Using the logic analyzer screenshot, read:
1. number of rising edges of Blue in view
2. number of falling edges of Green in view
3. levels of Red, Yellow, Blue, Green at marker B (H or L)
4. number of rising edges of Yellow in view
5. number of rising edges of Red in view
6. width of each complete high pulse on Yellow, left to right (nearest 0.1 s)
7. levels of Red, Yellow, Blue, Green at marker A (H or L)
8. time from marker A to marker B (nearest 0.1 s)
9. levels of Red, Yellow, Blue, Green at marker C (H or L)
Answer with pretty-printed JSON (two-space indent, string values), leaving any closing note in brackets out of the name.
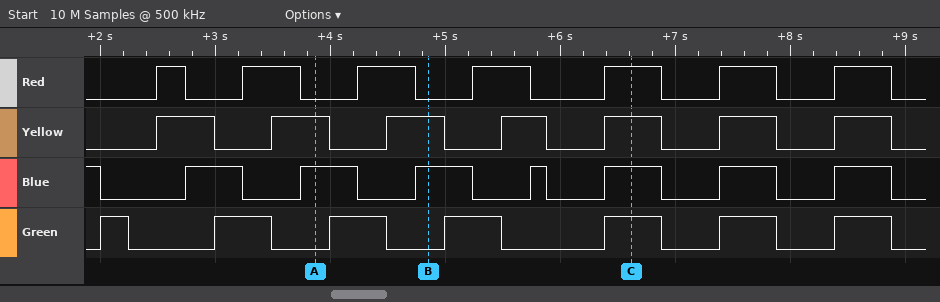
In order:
{
  "number of rising edges of Blue in view": "7",
  "number of falling edges of Green in view": "7",
  "levels of Red, Yellow, Blue, Green at marker B": "Red=L, Yellow=H, Blue=H, Green=L",
  "number of rising edges of Yellow in view": "7",
  "number of rising edges of Red in view": "7",
  "width of each complete high pulse on Yellow, left to right": "0.5 s, 0.5 s, 0.5 s, 0.4 s, 0.5 s, 0.5 s, 0.5 s",
  "levels of Red, Yellow, Blue, Green at marker A": "Red=L, Yellow=H, Blue=H, Green=L",
  "time from marker A to marker B": "1 s",
  "levels of Red, Yellow, Blue, Green at marker C": "Red=H, Yellow=H, Blue=H, Green=H"
}
